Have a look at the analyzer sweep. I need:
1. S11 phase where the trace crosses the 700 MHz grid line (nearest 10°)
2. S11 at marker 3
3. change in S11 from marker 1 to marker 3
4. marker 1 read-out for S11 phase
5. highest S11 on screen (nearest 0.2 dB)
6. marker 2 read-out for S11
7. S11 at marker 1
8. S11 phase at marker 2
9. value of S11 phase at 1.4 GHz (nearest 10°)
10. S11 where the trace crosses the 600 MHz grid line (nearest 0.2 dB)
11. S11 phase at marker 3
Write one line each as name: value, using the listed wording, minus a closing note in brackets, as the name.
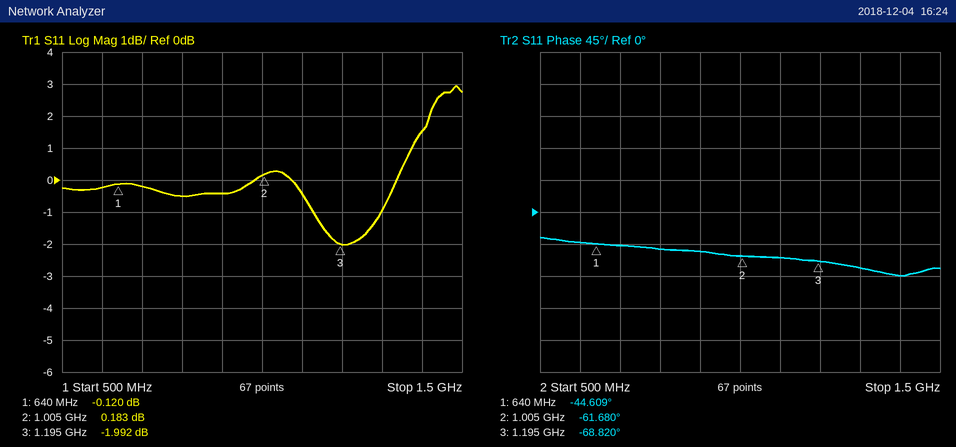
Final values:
S11 phase where the trace crosses the 700 MHz grid line: -50°
S11 at marker 3: -1.992 dB
change in S11 from marker 1 to marker 3: -1.872 dB
marker 1 read-out for S11 phase: -44.609°
highest S11 on screen: 3.0 dB
marker 2 read-out for S11: 0.183 dB
S11 at marker 1: -0.120 dB
S11 phase at marker 2: -61.680°
value of S11 phase at 1.4 GHz: -90°
S11 where the trace crosses the 600 MHz grid line: -0.2 dB
S11 phase at marker 3: -68.820°
